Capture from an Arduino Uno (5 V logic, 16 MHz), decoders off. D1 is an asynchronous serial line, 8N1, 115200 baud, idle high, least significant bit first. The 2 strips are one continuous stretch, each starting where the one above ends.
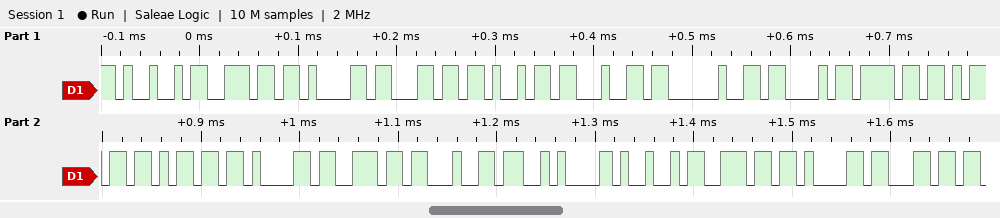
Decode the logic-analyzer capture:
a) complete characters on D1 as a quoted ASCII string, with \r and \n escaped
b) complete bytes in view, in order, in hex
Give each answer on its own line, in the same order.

"Inalid Command\nInal"
49 6E 61 6C 69 64 20 43 6F 6D 6D 61 6E 64 0A 49 6E 61 6C
